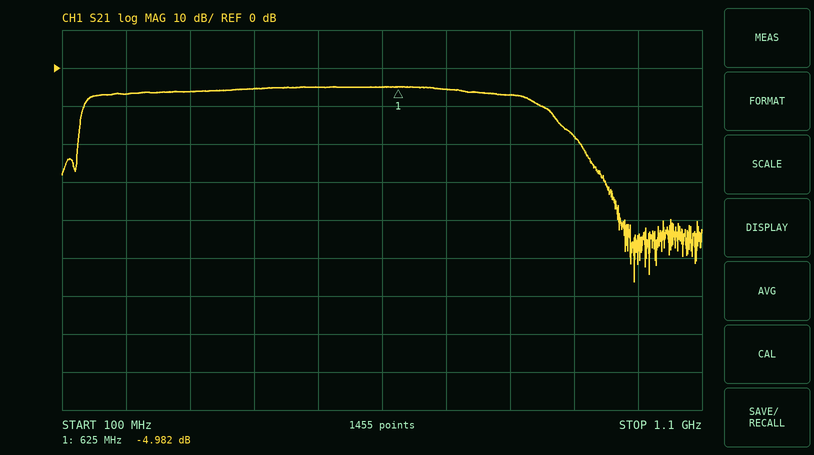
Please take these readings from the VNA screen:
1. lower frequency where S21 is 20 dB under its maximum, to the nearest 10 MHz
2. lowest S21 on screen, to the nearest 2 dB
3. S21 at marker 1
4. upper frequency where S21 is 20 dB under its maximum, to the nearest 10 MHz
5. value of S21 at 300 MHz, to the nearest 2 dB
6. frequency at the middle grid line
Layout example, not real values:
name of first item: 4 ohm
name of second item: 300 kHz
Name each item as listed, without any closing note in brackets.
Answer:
lower frequency where S21 is 20 dB under its maximum, to the nearest 10 MHz: 120 MHz
lowest S21 on screen, to the nearest 2 dB: -56 dB
S21 at marker 1: -4.982 dB
upper frequency where S21 is 20 dB under its maximum, to the nearest 10 MHz: 930 MHz
value of S21 at 300 MHz, to the nearest 2 dB: -6 dB
frequency at the middle grid line: 600 MHz
